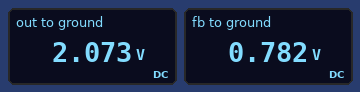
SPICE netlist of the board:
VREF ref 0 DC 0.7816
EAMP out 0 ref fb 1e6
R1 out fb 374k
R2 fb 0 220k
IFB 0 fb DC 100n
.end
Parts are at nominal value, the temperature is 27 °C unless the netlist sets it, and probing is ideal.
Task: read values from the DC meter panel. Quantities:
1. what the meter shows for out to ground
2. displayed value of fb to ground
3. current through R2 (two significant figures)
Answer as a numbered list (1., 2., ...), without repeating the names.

1. 2.073 V
2. 0.782 V
3. 3.6 µA
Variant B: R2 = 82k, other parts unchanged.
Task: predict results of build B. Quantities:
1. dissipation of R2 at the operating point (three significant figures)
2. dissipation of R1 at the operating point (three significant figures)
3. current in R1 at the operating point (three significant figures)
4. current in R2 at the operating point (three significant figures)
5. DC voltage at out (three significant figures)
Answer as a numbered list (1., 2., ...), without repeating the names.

1. 7.45 µW
2. 33.3 µW
3. 9.43 µA
4. 9.53 µA
5. 4.31 V
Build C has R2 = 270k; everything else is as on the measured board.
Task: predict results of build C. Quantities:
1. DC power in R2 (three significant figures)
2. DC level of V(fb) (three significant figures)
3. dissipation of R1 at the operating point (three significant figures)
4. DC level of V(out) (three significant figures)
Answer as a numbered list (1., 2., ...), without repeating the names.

1. 2.26 µW
2. 782 mV
3. 2.92 µW
4. 1.83 V
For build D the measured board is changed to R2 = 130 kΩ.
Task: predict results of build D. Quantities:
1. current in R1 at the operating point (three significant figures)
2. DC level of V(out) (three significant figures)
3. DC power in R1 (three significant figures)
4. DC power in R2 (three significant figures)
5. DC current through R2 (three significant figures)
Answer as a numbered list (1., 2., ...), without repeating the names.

1. 5.91 µA
2. 2.99 V
3. 13.1 µW
4. 4.70 µW
5. 6.01 µA
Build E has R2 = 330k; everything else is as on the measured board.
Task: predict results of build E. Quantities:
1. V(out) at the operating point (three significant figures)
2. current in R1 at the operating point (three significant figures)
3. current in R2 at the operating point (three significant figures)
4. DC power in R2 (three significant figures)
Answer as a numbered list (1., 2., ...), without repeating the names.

1. 1.63 V
2. 2.27 µA
3. 2.37 µA
4. 1.85 µW
